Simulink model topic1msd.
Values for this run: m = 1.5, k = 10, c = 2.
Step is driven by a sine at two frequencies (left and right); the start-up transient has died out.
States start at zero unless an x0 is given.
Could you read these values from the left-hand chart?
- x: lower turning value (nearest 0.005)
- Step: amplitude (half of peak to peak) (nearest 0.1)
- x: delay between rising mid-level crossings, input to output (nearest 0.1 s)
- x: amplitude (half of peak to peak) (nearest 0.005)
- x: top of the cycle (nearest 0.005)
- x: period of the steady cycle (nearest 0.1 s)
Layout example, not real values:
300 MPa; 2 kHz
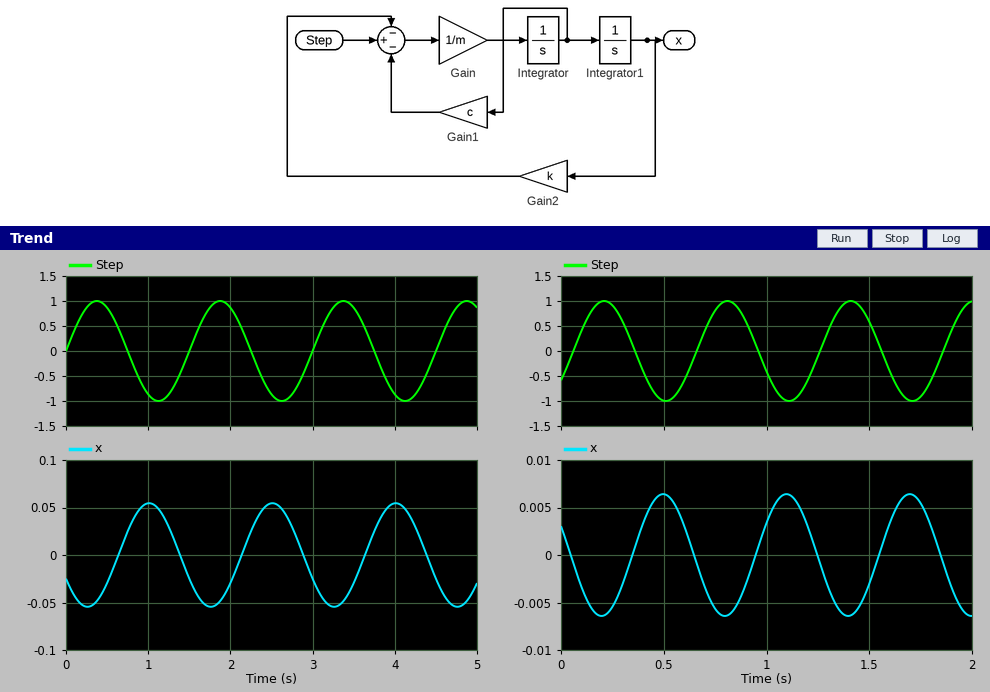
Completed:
-0.055; 1.0; 0.6 s; 0.055; 0.055; 1.5 s
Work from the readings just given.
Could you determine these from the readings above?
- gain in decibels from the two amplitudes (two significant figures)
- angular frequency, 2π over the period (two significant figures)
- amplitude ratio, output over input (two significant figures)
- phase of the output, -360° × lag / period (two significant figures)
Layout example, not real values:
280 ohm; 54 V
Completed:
-25 dB; 4.2 rad/s; 0.055; -140°
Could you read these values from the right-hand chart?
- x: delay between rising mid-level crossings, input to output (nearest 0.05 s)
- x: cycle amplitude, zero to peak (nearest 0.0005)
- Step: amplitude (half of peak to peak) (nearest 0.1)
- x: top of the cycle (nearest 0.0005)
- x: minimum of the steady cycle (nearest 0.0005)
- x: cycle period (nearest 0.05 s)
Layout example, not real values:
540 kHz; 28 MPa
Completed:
0.30 s; 0.0065; 1.0; 0.0065; -0.0065; 0.60 s
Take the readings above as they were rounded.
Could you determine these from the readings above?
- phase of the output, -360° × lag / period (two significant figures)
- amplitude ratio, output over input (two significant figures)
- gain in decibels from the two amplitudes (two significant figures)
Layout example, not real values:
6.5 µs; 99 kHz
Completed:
-180°; 0.0065; -44 dB
